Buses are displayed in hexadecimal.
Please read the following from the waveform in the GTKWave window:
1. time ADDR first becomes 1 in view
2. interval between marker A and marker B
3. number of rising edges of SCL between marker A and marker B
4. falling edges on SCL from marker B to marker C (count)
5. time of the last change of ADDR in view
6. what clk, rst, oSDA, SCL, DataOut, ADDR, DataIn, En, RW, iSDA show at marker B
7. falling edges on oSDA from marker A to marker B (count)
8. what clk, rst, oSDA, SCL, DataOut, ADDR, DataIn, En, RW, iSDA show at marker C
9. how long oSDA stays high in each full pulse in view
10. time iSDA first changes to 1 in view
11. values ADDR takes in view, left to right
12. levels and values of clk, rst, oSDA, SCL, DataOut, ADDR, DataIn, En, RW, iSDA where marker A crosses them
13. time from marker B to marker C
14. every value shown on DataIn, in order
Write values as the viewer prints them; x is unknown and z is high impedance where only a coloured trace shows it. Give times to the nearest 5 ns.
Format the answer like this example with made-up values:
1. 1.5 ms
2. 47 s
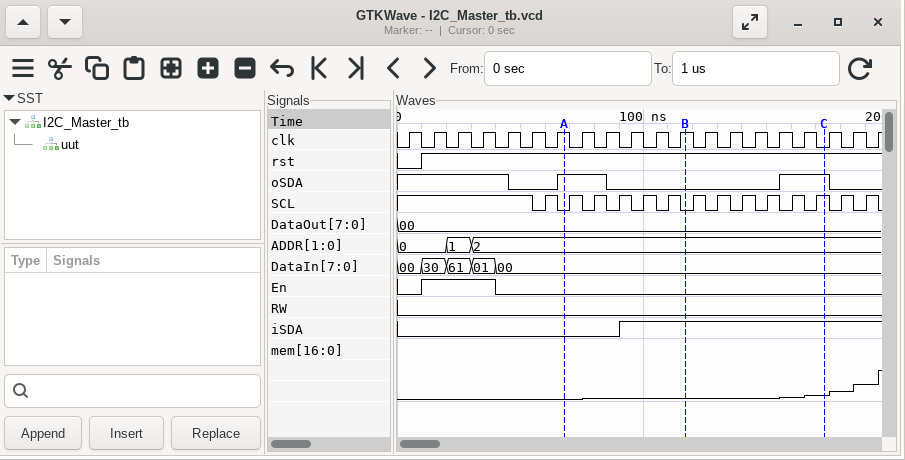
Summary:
1. 20 ns
2. 50 ns
3. 5
4. 5
5. 30 ns
6. clk=1, rst=1, oSDA=0, SCL=0, DataOut=00, ADDR=2, DataIn=00, En=0, RW=0, iSDA=1
7. 1
8. clk=0, rst=1, oSDA=1, SCL=1, DataOut=00, ADDR=2, DataIn=00, En=0, RW=0, iSDA=1
9. 20 ns, 20 ns
10. 90 ns
11. 0, 1, 2
12. clk=1, rst=1, oSDA=1, SCL=0, DataOut=00, ADDR=2, DataIn=00, En=0, RW=0, iSDA=0
13. 55 ns
14. 00, 30, 61, 01, 00
